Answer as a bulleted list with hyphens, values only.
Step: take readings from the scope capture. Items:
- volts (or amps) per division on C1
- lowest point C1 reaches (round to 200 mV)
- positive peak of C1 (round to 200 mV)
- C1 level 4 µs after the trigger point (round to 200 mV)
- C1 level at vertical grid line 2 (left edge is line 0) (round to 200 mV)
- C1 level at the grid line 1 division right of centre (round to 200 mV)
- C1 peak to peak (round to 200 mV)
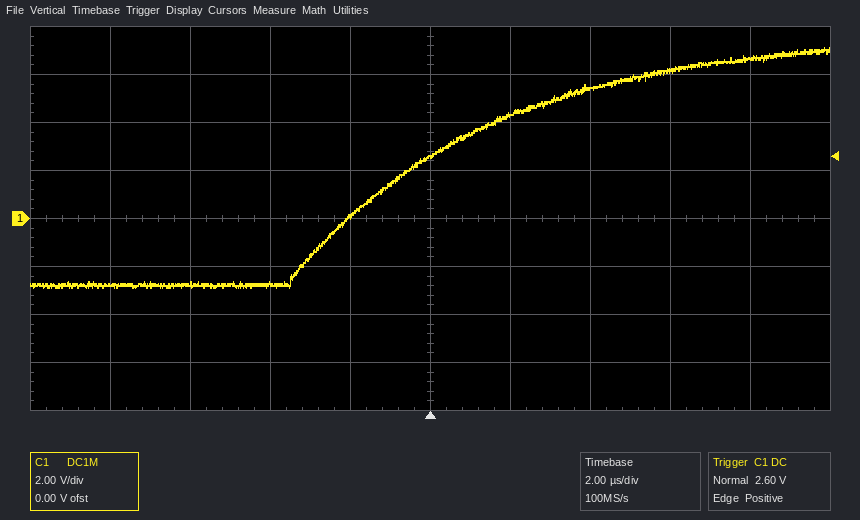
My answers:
- 2 V
- -2.8 V
- 7.2 V
- 5.4 V
- -2.8 V
- 4.2 V
- 10.0 V
